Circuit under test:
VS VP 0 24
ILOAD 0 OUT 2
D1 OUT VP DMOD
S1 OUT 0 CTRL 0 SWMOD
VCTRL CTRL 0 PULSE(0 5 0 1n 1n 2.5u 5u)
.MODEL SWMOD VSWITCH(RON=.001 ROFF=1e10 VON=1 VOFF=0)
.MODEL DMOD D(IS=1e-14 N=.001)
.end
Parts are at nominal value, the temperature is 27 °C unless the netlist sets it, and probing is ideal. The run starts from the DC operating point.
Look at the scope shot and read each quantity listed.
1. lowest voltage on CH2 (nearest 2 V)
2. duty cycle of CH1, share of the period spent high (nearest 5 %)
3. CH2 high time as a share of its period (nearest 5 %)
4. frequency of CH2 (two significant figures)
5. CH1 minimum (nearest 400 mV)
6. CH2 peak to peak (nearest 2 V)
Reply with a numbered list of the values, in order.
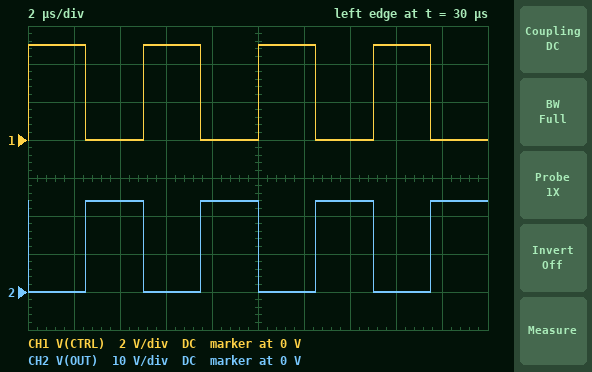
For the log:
1. 0 V
2. 50 %
3. 50 %
4. 200 kHz
5. 0 V
6. 24 V
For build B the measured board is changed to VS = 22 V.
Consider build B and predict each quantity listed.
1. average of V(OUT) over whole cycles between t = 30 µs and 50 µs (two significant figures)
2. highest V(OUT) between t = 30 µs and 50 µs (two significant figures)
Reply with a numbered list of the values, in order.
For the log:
1. 11 V
2. 22 V
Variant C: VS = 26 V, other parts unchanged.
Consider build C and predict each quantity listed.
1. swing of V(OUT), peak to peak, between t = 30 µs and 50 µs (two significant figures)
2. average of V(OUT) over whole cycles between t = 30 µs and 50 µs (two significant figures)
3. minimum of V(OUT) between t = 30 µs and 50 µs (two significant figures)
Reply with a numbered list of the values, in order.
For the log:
1. 26 V
2. 13 V
3. 2.0 mV
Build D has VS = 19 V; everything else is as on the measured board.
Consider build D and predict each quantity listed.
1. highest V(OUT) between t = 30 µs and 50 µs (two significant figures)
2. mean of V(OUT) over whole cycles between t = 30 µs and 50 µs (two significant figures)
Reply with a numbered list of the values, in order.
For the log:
1. 19 V
2. 9.5 V
